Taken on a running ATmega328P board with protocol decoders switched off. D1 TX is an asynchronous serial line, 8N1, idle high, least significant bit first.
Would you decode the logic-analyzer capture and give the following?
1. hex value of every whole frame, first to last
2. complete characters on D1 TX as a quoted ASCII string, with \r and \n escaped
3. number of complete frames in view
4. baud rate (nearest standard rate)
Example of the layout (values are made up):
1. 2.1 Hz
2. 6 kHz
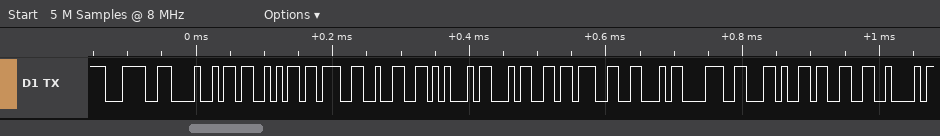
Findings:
1. 0x3C 0x48 0x53 0x3B 0x32 0x45 0x34 0x3B 0x46 0x38 0x2C 0x33 0x42
2. "<HS;2E4;F8,3B"
3. 13
4. 115200 baud
